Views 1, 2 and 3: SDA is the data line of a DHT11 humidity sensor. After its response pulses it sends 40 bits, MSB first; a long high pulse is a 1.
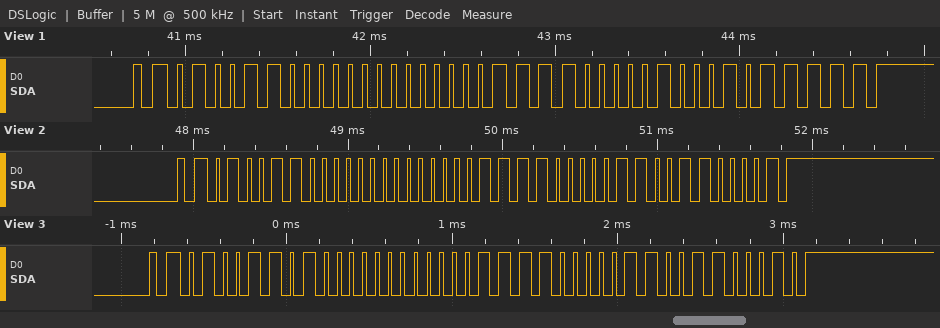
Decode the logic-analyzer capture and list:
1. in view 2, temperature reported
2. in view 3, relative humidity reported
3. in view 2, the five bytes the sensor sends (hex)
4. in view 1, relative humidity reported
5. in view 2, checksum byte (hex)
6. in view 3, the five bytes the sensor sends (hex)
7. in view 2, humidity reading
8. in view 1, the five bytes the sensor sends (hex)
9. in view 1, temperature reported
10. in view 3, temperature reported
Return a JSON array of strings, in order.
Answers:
["15.6 °C", "77 %", "4C 00 0F 06 61", "76 %", "0x61", "4D 00 0F 06 62", "76 %", "4C 00 0F 04 5F", "15.4 °C", "15.6 °C"]
